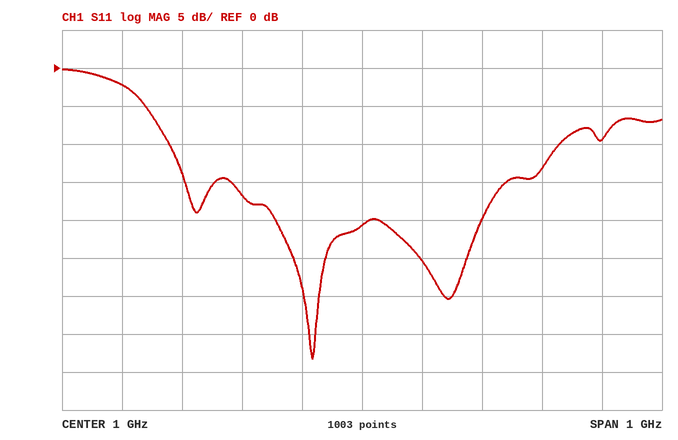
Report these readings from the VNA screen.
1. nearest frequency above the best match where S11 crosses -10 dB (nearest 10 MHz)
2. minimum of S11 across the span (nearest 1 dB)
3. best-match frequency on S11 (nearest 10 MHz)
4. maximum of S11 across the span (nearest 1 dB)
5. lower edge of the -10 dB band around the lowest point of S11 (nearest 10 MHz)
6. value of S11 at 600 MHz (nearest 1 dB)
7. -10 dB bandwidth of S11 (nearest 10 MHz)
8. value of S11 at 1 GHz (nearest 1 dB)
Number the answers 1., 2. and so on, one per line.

1. 1.33 GHz
2. -38 dB
3. 920 MHz
4. 0 dB
5. 680 MHz
6. -2 dB
7. 650 MHz
8. -21 dB
